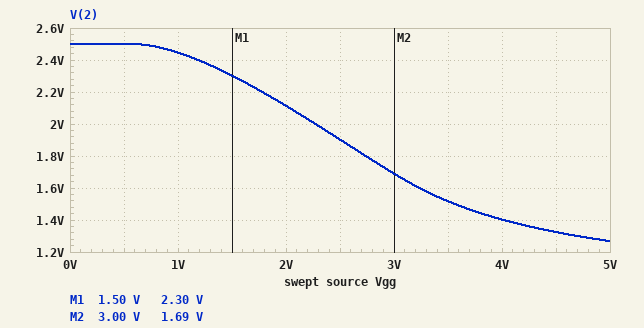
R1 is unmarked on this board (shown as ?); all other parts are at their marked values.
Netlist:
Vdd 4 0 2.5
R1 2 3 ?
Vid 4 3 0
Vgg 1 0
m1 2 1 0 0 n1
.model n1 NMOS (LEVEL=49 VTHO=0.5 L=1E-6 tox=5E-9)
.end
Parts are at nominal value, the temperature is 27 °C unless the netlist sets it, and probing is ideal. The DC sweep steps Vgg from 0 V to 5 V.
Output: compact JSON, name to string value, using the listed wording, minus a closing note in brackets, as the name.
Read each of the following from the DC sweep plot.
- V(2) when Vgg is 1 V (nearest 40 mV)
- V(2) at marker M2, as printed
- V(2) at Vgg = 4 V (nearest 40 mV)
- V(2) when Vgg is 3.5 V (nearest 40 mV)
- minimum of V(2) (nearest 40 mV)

{"V(2) when Vgg is 1 V": "2.44 V", "V(2) at marker M2, as printed": "1.69 V", "V(2) at Vgg = 4 V": "1.40 V", "V(2) when Vgg is 3.5 V": "1.52 V", "minimum of V(2)": "1.28 V"}
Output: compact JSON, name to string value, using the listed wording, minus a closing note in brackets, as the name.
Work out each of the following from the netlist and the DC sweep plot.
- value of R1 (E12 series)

{"value of R1": "560 Ω"}
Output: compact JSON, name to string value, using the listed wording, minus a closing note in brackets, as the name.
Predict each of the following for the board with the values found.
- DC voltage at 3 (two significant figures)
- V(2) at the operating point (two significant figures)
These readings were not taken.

{"DC voltage at 3": "2.5 V", "V(2) at the operating point": "2.5 V"}
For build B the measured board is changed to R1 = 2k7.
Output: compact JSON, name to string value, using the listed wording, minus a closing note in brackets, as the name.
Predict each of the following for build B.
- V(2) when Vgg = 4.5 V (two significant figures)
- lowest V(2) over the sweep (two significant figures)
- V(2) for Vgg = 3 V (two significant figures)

{"V(2) when Vgg = 4.5 V": "380 mV", "lowest V(2) over the sweep": "360 mV", "V(2) for Vgg = 3 V": "480 mV"}
